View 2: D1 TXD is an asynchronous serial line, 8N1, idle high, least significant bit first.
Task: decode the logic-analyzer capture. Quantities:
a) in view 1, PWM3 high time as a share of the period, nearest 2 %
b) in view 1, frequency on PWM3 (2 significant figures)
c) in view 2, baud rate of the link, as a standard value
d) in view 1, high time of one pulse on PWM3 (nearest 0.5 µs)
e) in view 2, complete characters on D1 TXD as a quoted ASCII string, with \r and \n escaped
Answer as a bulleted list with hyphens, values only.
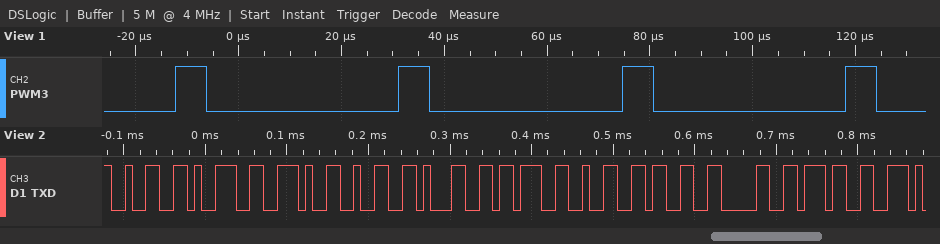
- 14 %
- 23 kHz
- 115200 baud
- 6.0 µs
- "29.21;2307"
